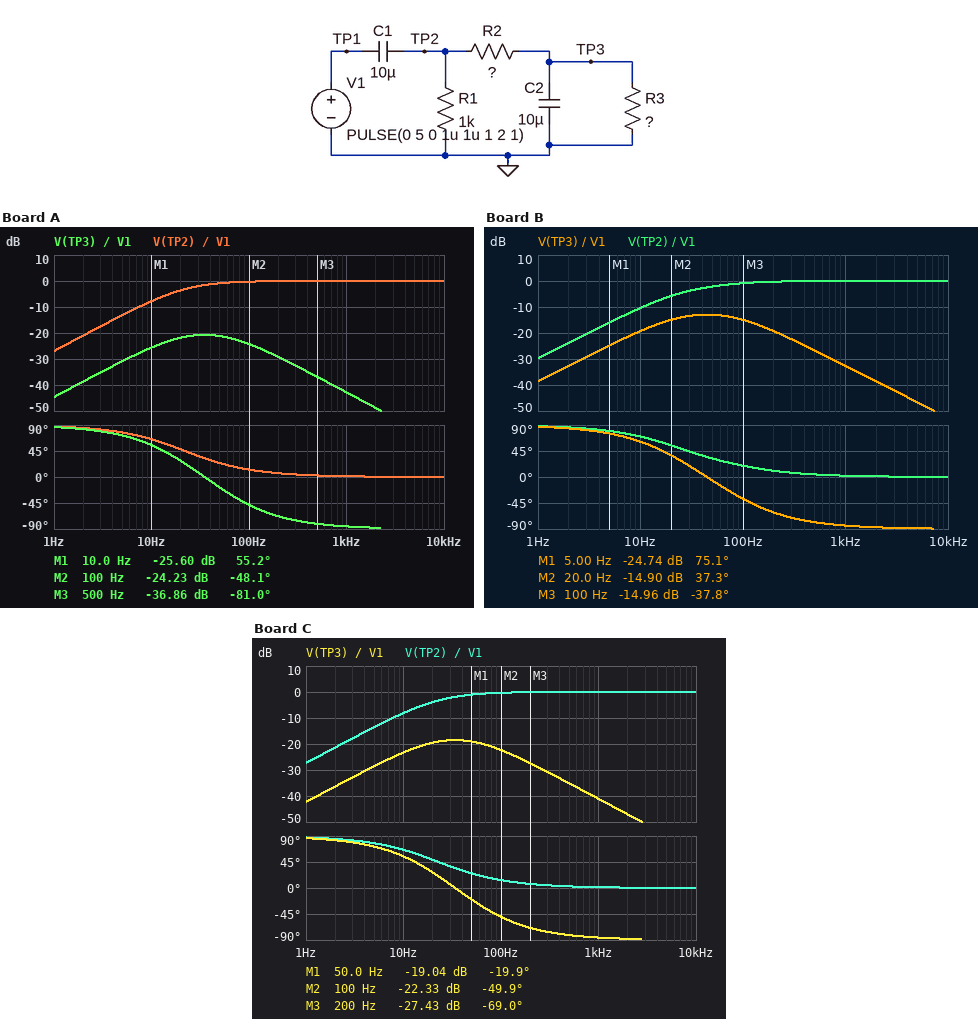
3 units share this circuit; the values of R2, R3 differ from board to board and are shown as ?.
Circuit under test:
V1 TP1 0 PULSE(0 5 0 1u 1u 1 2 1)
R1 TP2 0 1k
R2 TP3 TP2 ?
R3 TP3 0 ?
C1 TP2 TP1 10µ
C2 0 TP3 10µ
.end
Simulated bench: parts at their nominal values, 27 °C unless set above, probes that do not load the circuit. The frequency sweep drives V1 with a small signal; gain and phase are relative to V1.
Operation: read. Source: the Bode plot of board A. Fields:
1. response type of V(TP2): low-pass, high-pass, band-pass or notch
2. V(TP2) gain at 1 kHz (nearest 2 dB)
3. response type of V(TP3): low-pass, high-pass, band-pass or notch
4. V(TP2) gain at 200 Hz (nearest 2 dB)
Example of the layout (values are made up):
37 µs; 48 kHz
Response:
high-pass; 0 dB; band-pass; 0 dB
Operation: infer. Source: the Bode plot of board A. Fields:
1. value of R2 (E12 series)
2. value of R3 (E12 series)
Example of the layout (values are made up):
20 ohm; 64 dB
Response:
2.2 kΩ; 330 Ω
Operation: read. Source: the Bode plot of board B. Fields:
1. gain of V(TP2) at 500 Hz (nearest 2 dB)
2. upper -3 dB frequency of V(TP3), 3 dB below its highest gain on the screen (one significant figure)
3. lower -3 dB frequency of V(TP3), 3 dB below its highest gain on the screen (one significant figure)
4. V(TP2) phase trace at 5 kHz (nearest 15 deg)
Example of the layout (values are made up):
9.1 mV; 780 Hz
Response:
0 dB; 100 Hz; 20 Hz; 0 deg
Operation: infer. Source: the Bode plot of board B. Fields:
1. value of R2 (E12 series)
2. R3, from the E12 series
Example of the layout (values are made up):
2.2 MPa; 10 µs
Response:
680 Ω; 390 Ω
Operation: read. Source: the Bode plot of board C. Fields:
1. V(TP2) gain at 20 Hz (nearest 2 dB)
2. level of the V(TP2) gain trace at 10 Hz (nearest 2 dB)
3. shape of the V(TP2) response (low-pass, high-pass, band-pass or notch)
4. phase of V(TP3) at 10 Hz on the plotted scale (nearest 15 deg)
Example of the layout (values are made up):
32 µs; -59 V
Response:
-4 dB; -8 dB; high-pass; 60 deg
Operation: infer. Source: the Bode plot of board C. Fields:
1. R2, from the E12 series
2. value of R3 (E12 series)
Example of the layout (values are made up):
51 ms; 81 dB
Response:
1.8 kΩ; 390 Ω
